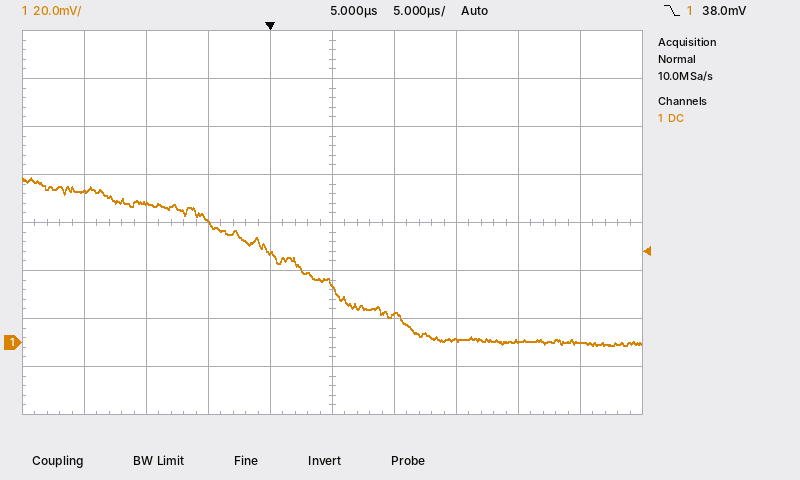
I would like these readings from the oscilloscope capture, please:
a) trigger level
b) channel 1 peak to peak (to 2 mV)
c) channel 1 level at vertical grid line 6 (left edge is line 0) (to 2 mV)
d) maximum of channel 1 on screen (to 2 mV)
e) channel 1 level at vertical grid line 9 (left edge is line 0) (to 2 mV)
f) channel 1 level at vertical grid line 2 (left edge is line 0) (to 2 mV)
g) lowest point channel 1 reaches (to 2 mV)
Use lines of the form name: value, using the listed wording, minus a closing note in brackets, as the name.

trigger level: 38.0 mV
channel 1 peak to peak: 70 mV
channel 1 level at vertical grid line 6 (left edge is line 0): 12 mV
maximum of channel 1 on screen: 68 mV
channel 1 level at vertical grid line 9 (left edge is line 0): 0 mV
channel 1 level at vertical grid line 2 (left edge is line 0): 58 mV
lowest point channel 1 reaches: -2 mV
